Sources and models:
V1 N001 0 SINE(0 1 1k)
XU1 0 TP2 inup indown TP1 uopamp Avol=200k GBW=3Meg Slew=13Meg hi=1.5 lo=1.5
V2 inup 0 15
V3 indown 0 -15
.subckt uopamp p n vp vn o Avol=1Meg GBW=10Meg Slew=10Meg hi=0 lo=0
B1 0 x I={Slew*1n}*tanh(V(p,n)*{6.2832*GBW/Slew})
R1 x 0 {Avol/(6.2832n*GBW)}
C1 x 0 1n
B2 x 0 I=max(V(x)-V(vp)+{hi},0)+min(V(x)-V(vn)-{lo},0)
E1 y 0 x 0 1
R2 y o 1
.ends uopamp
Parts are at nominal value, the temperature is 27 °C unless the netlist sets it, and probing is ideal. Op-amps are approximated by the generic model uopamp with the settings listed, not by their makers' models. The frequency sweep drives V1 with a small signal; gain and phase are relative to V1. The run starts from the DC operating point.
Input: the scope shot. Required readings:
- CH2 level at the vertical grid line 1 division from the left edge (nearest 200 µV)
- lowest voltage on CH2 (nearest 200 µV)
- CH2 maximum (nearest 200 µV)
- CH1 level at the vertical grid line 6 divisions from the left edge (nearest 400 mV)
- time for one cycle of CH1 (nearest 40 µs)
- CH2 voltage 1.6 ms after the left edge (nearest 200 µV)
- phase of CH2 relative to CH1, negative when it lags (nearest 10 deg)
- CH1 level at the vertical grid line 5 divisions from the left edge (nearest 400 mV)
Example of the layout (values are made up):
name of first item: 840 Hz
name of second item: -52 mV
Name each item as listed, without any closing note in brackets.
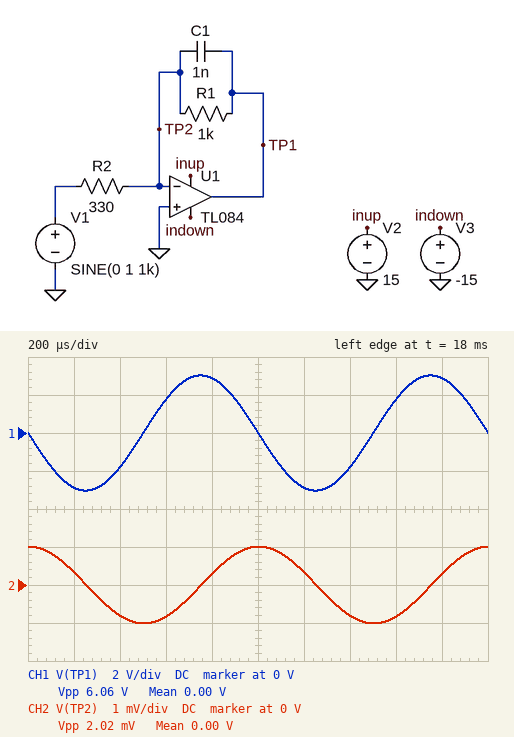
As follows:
CH2 level at the vertical grid line 1 division from the left edge: 400 µV
lowest voltage on CH2: -1.0 mV
CH2 maximum: 1.0 mV
CH1 level at the vertical grid line 6 divisions from the left edge: -2.8 V
time for one cycle of CH1: 1.00 ms
CH2 voltage 1.6 ms after the left edge: -800 µV
phase of CH2 relative to CH1, negative when it lags: -90 deg
CH1 level at the vertical grid line 5 divisions from the left edge: 0 V
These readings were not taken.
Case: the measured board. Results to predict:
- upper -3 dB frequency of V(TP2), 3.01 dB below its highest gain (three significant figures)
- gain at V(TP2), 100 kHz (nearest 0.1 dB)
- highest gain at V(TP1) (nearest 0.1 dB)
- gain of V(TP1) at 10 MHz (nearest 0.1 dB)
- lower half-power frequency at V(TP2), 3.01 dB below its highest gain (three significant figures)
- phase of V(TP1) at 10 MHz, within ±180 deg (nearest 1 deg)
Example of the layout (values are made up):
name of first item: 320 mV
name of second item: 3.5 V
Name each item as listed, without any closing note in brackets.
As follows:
upper -3 dB frequency of V(TP2), 3.01 dB below its highest gain: 3.76 MHz
gain at V(TP2), 100 kHz: -21.8 dB
highest gain at V(TP1): 9.6 dB
gain of V(TP1) at 10 MHz: -35.7 dB
lower half-power frequency at V(TP2), 3.01 dB below its highest gain: 127 kHz
phase of V(TP1) at 10 MHz, within ±180 deg: 20 deg
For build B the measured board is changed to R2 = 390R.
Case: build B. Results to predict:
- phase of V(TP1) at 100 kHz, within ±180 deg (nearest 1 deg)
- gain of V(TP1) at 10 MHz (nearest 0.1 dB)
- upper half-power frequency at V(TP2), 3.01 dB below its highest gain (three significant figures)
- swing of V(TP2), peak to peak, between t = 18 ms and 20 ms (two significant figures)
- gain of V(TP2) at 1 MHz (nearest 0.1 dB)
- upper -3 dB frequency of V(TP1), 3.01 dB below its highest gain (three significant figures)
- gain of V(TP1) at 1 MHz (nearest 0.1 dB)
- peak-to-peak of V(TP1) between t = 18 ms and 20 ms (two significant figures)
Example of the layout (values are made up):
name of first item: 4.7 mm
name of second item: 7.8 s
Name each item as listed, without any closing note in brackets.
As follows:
phase of V(TP1) at 100 kHz, within ±180 deg: 143 deg
gain of V(TP1) at 10 MHz: -37.1 dB
upper half-power frequency at V(TP2), 3.01 dB below its highest gain: 3.69 MHz
swing of V(TP2), peak to peak, between t = 18 ms and 20 ms: 1.7 mV
gain of V(TP2) at 1 MHz: -18.9 dB
upper -3 dB frequency of V(TP1), 3.01 dB below its highest gain: 139 kHz
gain of V(TP1) at 1 MHz: -9.4 dB
peak-to-peak of V(TP1) between t = 18 ms and 20 ms: 5.1 V
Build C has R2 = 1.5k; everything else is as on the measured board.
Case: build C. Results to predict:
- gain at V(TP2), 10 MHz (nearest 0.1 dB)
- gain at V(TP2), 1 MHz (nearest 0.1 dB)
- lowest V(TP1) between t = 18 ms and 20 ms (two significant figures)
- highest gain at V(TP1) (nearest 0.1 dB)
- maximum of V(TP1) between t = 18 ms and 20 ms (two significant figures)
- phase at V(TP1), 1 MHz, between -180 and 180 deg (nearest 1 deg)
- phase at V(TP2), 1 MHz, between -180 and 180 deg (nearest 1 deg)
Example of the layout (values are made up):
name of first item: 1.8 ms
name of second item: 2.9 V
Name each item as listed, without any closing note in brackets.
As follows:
gain at V(TP2), 10 MHz: -39.9 dB
gain at V(TP2), 1 MHz: -29.9 dB
lowest V(TP1) between t = 18 ms and 20 ms: -670 mV
highest gain at V(TP1): -3.5 dB
maximum of V(TP1) between t = 18 ms and 20 ms: 670 mV
phase at V(TP1), 1 MHz, between -180 and 180 deg: 81 deg
phase at V(TP2), 1 MHz, between -180 and 180 deg: -9 deg
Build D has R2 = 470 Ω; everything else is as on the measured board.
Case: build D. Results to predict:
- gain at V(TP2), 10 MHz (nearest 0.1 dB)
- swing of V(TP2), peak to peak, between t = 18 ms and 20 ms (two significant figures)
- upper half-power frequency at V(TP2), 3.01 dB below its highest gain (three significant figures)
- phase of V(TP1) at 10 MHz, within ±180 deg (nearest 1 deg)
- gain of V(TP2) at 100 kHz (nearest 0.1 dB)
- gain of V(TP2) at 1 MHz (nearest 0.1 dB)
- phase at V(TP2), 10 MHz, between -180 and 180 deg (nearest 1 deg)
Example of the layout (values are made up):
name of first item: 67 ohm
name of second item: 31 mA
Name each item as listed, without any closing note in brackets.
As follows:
gain at V(TP2), 10 MHz: -29.9 dB
swing of V(TP2), peak to peak, between t = 18 ms and 20 ms: 1.4 mV
upper half-power frequency at V(TP2), 3.01 dB below its highest gain: 3.62 MHz
phase of V(TP1) at 10 MHz, within ±180 deg: 19 deg
gain of V(TP2) at 100 kHz: -24.7 dB
gain of V(TP2) at 1 MHz: -20.4 dB
phase at V(TP2), 10 MHz, between -180 and 180 deg: -67 deg
